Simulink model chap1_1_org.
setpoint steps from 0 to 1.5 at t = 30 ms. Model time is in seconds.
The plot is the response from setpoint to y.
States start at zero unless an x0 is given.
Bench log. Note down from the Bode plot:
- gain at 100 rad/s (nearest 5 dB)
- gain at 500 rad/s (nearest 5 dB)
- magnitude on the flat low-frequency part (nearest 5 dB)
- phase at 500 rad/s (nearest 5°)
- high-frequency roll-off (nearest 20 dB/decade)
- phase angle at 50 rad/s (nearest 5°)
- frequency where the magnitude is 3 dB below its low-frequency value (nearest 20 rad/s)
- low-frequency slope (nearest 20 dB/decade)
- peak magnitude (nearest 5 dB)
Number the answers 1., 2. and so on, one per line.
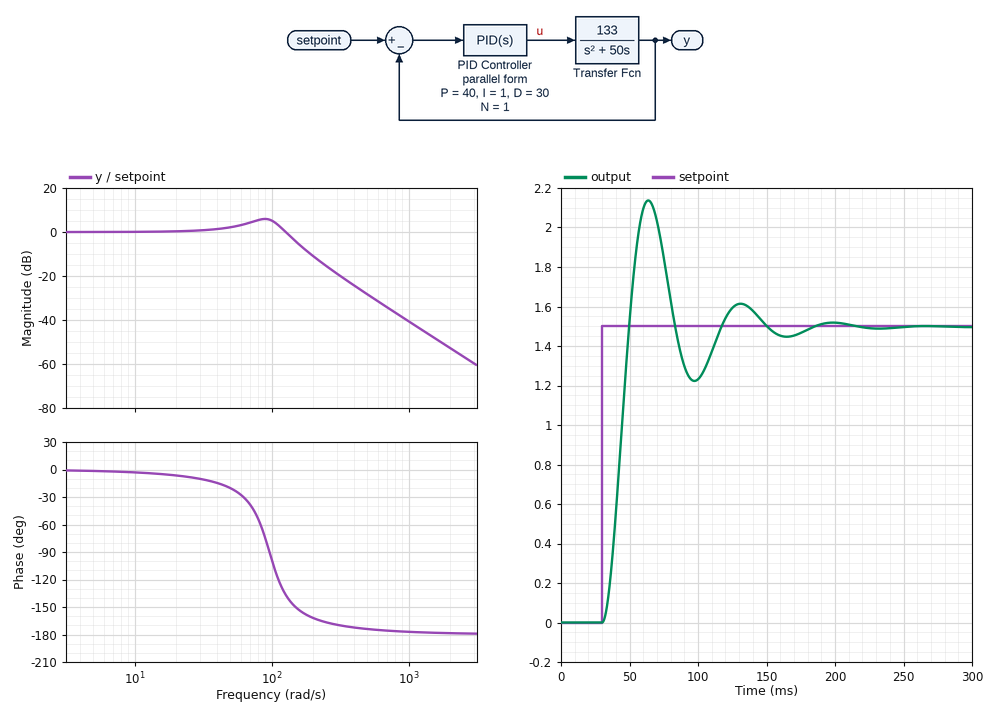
1. 5 dB
2. -30 dB
3. 0 dB
4. -175°
5. -40 dB/decade
6. -20°
7. 140 rad/s
8. 0 dB/decade
9. 5 dB
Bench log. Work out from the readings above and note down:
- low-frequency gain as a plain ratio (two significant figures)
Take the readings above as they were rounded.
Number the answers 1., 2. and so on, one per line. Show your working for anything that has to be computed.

1. 10^(0 / 20) = 1.0
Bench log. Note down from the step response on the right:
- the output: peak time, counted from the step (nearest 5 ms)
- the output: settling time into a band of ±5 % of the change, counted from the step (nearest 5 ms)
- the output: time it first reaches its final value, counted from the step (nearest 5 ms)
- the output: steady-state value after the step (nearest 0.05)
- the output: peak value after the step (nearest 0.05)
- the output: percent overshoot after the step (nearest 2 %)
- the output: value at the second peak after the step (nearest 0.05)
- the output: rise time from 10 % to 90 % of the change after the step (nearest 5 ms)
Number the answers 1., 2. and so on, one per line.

1. 35 ms
2. 110 ms
3. 20 ms
4. 1.50
5. 2.15
6. 42 %
7. 1.60
8. 15 ms
